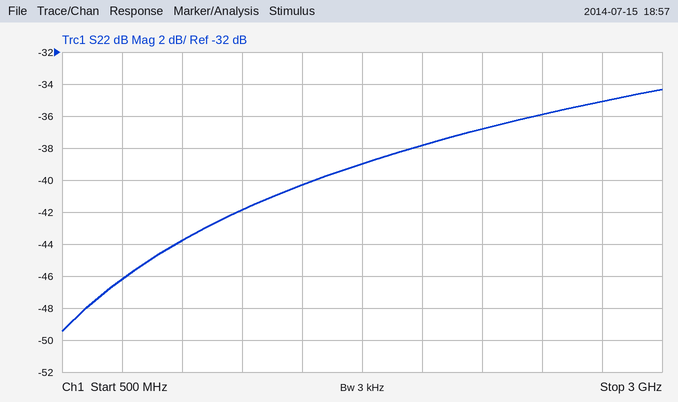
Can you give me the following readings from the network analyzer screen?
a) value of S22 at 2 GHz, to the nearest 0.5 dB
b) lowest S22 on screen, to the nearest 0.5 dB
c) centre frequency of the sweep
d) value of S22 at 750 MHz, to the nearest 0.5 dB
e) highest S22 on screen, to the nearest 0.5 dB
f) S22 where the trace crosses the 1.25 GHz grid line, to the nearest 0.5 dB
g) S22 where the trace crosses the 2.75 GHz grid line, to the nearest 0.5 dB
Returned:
-38.0 dB
-49.5 dB
1.75 GHz
-46.0 dB
-34.5 dB
-42.0 dB
-35.0 dB
